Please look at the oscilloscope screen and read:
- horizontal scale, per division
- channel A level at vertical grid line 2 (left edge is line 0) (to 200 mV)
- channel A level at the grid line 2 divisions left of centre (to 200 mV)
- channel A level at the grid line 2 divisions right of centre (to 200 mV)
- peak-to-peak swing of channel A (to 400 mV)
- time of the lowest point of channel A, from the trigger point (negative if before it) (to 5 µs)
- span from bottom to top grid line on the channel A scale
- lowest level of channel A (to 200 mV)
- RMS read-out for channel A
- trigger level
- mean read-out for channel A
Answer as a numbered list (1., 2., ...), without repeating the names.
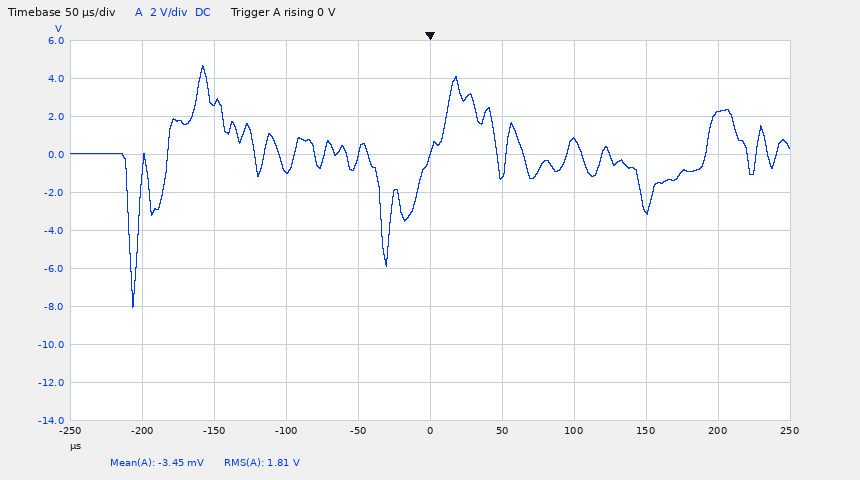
1. 50 µs
2. 2.8 V
3. -800 mV
4. 800 mV
5. 12.8 V
6. -205 µs
7. 20 V
8. -8.0 V
9. 1.81 V
10. 0 V
11. -3.45 mV
